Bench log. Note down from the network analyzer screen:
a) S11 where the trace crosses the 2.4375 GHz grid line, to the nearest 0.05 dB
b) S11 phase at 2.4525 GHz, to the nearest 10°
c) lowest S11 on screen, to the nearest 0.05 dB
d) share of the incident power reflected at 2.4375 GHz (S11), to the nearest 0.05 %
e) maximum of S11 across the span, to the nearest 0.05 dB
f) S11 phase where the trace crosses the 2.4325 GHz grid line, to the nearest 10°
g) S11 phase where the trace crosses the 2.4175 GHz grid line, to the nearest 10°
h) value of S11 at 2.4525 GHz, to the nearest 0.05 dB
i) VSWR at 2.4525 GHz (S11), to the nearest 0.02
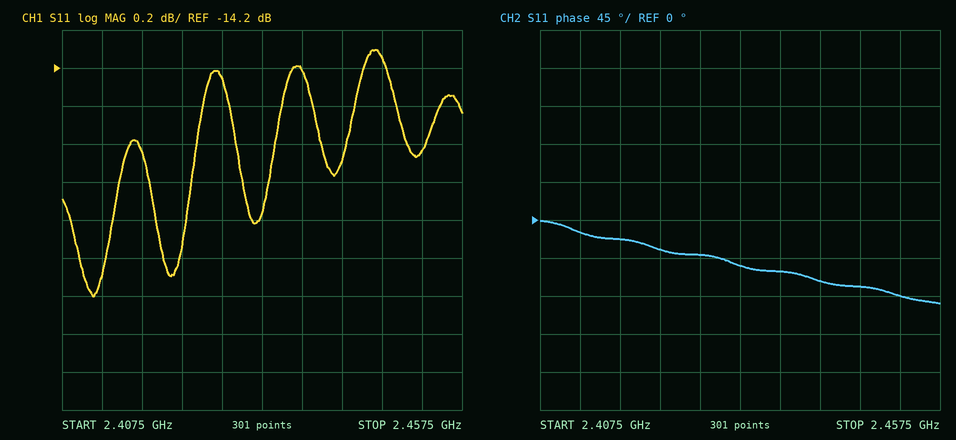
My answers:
-14.20 dB
-90°
-15.40 dB
3.80 %
-14.10 dB
-50°
-20°
-14.65 dB
1.46
